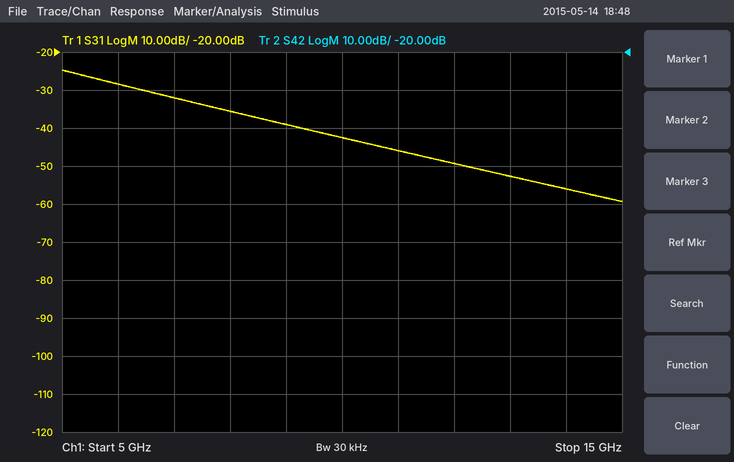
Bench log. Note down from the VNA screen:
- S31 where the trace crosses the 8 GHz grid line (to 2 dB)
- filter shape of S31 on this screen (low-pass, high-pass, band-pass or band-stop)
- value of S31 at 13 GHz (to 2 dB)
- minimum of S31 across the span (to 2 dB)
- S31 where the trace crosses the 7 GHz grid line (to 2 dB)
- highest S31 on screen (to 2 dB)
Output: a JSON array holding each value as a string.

["-36 dB", "low-pass", "-52 dB", "-60 dB", "-32 dB", "-24 dB"]
